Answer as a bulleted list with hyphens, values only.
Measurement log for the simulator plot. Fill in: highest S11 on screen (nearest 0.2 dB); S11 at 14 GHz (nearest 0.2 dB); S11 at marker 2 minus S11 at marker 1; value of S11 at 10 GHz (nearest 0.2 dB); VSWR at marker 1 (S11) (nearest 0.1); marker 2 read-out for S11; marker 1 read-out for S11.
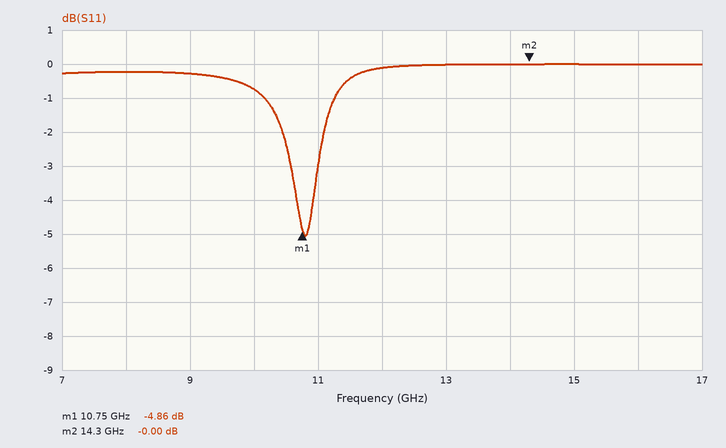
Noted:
- 0.0 dB
- 0.0 dB
- 4.86 dB
- -0.8 dB
- 3.7
- -0.00 dB
- -4.86 dB
